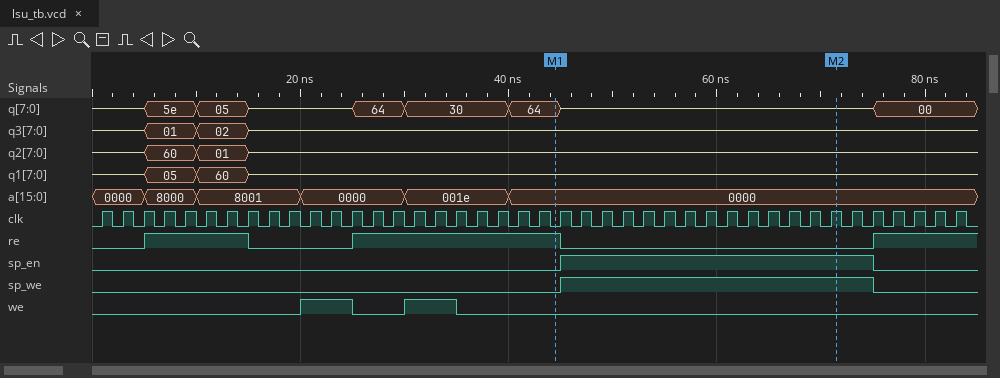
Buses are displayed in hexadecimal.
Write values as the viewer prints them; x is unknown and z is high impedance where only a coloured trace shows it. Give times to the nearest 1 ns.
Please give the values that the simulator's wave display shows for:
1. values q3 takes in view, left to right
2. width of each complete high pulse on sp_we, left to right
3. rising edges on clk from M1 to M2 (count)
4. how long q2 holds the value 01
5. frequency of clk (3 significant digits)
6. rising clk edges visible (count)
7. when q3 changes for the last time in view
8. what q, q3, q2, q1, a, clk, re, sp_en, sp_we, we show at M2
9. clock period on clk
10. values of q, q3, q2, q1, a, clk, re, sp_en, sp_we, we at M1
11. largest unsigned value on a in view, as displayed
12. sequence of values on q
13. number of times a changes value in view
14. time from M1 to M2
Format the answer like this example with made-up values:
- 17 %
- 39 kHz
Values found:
- z, 01, 02, z
- 30 ns
- 14
- 5 ns
- 500 MHz
- 42
- 15 ns
- q=z, q3=z, q2=z, q1=z, a=0000, clk=1, re=0, sp_en=1, sp_we=1, we=0
- 2 ns
- q=64, q3=z, q2=z, q1=z, a=0000, clk=0, re=1, sp_en=0, sp_we=0, we=0
- 8001
- z, 5e, 05, z, 64, 30, 64, z, 00
- 5
- 27 ns
